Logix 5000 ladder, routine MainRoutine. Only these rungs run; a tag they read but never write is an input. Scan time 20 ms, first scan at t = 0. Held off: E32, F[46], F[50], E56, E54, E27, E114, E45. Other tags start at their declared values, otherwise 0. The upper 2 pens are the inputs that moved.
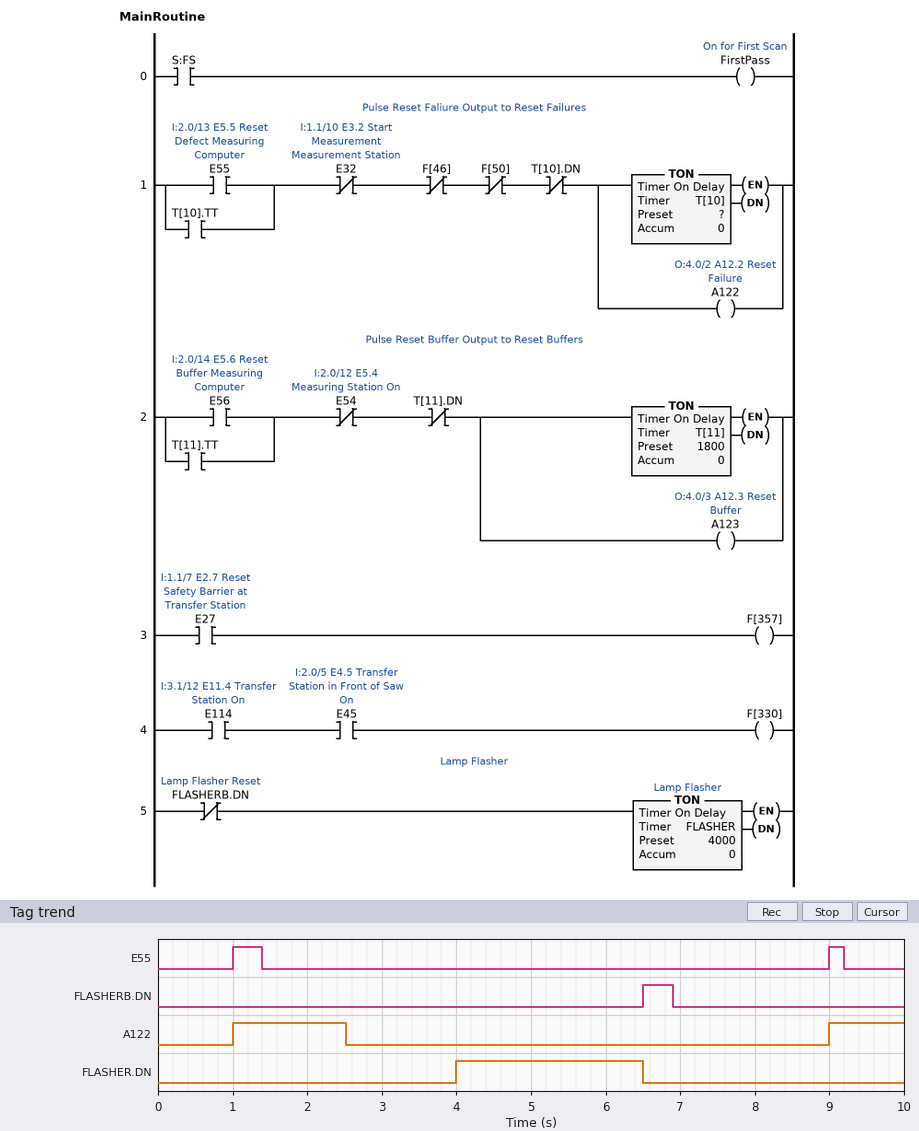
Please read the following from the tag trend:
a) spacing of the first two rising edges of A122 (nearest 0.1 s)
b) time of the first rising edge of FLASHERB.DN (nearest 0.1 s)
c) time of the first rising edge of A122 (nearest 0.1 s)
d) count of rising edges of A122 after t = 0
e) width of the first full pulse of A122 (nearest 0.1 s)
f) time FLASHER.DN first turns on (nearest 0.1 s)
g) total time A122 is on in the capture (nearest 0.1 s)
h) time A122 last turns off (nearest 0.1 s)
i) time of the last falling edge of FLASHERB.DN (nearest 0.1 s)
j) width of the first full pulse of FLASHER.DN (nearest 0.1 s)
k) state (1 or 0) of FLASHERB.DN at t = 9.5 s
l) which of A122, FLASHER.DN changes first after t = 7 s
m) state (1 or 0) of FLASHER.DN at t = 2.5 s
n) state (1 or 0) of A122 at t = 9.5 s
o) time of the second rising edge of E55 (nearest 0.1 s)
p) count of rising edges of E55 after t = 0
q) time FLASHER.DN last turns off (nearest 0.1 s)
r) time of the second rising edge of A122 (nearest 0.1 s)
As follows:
8.0 s
6.5 s
1.0 s
2
1.5 s
4.0 s
2.5 s
2.5 s
6.9 s
2.5 s
0
A122
0
1
9.0 s
2
6.5 s
9.0 s
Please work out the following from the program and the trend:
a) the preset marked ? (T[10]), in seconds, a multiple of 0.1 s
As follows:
1.5 s
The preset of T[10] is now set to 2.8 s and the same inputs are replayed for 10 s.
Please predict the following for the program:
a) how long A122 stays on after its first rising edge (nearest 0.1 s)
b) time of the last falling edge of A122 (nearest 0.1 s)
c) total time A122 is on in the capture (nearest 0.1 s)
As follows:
2.8 s
3.8 s
3.8 s
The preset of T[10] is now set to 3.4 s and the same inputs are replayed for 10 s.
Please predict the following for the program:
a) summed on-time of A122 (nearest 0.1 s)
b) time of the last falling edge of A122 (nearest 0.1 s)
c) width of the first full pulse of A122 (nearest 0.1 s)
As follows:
4.4 s
4.4 s
3.4 s
